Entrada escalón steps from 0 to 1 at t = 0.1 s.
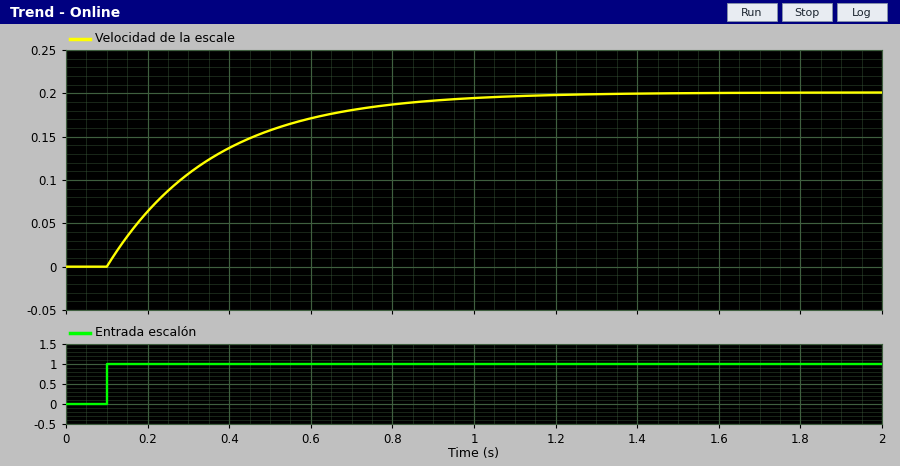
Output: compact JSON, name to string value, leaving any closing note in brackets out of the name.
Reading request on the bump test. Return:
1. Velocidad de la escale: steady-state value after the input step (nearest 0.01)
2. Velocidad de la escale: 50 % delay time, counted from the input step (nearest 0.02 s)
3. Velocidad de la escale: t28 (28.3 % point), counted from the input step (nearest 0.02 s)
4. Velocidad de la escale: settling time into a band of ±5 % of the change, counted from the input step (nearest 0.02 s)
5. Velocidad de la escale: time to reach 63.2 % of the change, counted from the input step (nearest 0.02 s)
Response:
{"Velocidad de la escale: steady-state value after the input step": "0.20", "Velocidad de la escale: 50 % delay time, counted from the input step": "0.18 s", "Velocidad de la escale: t28 (28.3 % point), counted from the input step": "0.08 s", "Velocidad de la escale: settling time into a band of ±5 % of the change, counted from the input step": "0.78 s", "Velocidad de la escale: time to reach 63.2 % of the change, counted from the input step": "0.26 s"}
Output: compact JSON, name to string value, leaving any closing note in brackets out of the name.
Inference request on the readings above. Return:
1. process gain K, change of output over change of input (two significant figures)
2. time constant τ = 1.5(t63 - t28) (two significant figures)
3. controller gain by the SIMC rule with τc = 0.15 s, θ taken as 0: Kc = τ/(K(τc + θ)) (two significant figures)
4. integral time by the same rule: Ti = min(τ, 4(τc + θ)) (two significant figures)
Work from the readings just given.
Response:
{"process gain K, change of output over change of input": "0.20", "time constant τ = 1.5(t63 - t28)": "0.27 s", "controller gain by the SIMC rule with τc = 0.15 s, θ taken as 0: Kc = τ/(K(τc + θ))": "9.0", "integral time by the same rule: Ti = min(τ, 4(τc + θ))": "0.27 s"}
